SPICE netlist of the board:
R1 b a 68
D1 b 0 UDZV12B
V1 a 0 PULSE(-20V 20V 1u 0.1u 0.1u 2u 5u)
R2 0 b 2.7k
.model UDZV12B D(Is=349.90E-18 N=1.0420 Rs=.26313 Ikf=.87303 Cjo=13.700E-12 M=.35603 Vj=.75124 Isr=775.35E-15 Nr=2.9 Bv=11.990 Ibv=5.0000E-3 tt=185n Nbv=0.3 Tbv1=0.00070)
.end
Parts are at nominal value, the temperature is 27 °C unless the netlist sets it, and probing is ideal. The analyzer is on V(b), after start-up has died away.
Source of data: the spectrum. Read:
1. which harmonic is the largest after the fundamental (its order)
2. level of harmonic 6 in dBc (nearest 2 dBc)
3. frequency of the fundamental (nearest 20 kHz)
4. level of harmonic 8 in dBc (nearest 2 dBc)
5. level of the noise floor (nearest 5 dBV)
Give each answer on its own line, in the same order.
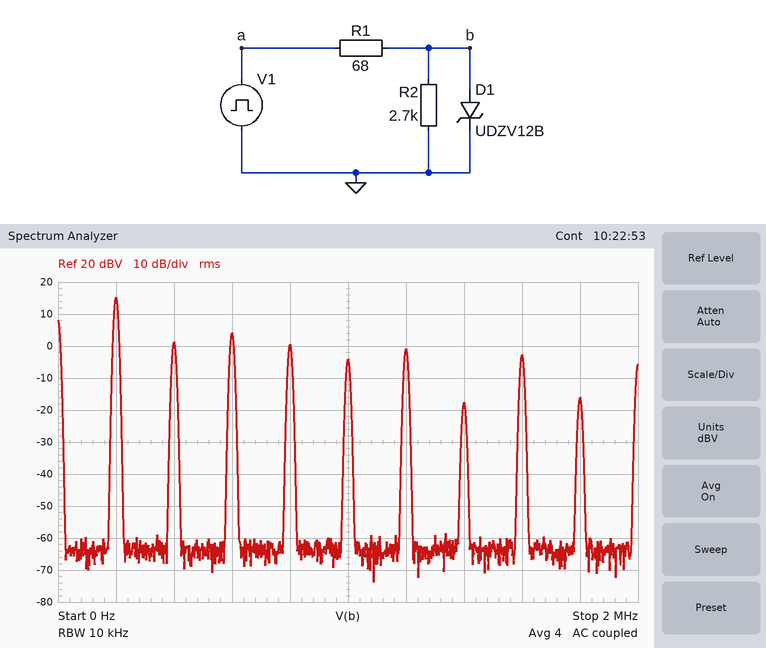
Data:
3
-16 dBc
200 kHz
-18 dBc
-65 dBV
